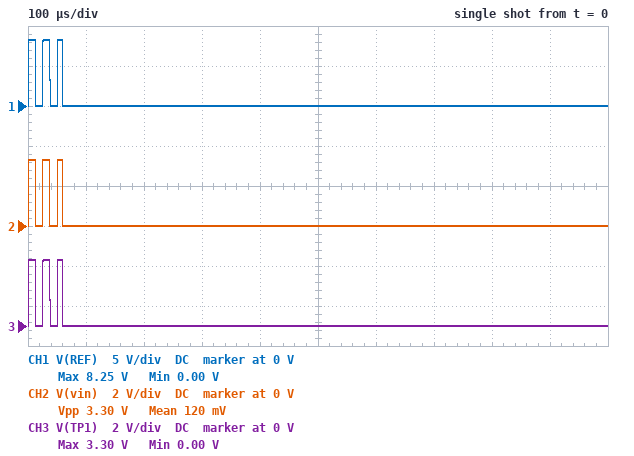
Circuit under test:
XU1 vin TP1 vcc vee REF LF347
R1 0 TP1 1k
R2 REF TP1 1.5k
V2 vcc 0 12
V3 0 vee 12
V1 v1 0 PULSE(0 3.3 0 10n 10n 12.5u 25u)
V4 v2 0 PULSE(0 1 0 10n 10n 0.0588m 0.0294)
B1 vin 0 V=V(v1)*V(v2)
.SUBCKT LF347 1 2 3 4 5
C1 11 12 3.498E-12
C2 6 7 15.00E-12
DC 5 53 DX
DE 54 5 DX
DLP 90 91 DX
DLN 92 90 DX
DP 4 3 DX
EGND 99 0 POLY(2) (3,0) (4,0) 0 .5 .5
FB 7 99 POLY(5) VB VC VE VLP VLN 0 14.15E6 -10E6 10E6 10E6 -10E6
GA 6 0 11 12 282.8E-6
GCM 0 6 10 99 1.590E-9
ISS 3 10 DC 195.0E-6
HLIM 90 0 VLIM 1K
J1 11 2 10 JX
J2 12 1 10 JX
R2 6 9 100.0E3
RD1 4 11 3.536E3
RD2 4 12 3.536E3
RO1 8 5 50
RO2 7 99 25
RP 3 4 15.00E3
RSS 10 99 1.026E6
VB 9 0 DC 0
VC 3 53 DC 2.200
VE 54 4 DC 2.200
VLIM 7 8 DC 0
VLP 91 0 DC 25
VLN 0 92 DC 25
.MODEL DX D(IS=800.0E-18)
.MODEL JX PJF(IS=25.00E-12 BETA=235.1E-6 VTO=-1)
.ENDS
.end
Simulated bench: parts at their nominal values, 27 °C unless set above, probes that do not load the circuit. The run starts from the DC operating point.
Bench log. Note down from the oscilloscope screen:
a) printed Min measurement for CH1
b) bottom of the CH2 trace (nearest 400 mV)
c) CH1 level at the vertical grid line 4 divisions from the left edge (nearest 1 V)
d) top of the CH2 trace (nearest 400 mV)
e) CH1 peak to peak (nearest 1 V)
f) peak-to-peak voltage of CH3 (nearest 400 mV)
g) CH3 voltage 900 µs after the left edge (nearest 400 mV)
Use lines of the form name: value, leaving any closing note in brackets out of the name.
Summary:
printed Min measurement for CH1: 0.00 V
bottom of the CH2 trace: 0 V
CH1 level at the vertical grid line 4 divisions from the left edge: 0 V
top of the CH2 trace: 3.2 V
CH1 peak to peak: 8 V
peak-to-peak voltage of CH3: 3.2 V
CH3 voltage 900 µs after the left edge: 0 V
